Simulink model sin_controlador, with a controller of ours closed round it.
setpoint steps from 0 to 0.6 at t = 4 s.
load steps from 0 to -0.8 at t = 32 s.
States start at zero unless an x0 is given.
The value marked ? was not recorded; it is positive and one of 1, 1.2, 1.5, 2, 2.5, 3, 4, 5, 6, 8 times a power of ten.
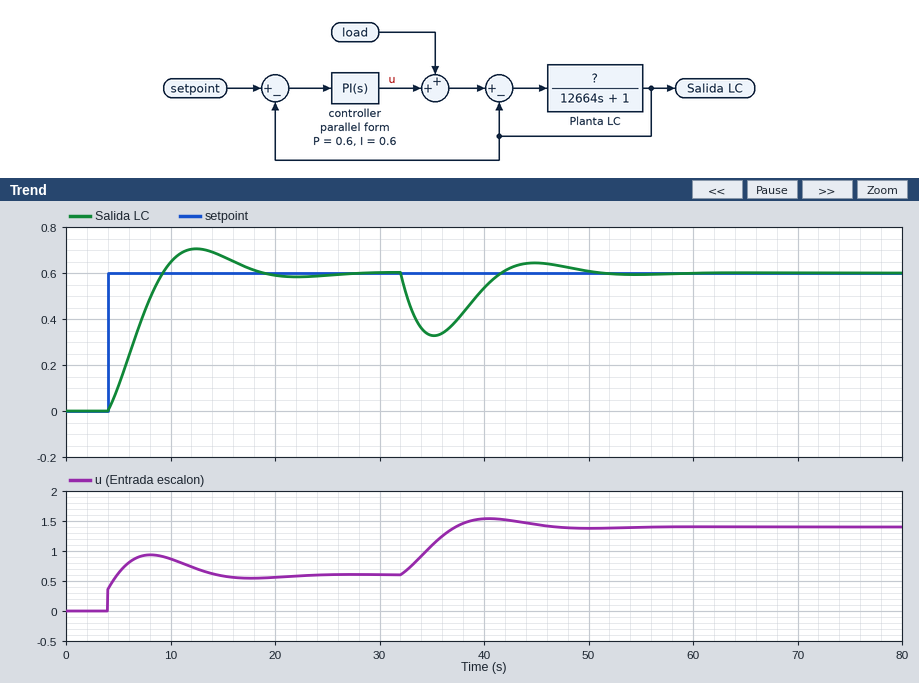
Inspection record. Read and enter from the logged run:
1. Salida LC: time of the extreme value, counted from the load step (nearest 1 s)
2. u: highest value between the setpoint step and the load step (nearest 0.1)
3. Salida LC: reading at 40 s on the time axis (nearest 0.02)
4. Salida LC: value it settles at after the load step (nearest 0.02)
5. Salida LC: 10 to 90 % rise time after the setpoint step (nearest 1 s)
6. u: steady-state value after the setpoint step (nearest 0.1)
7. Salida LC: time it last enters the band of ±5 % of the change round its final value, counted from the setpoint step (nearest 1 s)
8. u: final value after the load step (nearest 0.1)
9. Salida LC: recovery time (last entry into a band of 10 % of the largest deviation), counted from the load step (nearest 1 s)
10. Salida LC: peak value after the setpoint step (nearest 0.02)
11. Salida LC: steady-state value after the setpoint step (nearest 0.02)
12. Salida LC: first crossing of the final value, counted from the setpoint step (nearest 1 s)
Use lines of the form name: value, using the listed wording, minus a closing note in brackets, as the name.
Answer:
Salida LC: time of the extreme value, counted from the load step: 3 s
u: highest value between the setpoint step and the load step: 0.9
Salida LC: reading at 40 s on the time axis: 0.54
Salida LC: value it settles at after the load step: 0.60
Salida LC: 10 to 90 % rise time after the setpoint step: 4 s
u: steady-state value after the setpoint step: 0.6
Salida LC: time it last enters the band of ±5 % of the change round its final value, counted from the setpoint step: 13 s
u: final value after the load step: 1.4
Salida LC: recovery time (last entry into a band of 10 % of the largest deviation), counted from the load step: 16 s
Salida LC: peak value after the setpoint step: 0.70
Salida LC: steady-state value after the setpoint step: 0.60
Salida LC: first crossing of the final value, counted from the setpoint step: 5 s
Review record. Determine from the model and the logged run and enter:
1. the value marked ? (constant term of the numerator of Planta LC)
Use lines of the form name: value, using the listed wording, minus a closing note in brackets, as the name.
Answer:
the value marked ?: 3000
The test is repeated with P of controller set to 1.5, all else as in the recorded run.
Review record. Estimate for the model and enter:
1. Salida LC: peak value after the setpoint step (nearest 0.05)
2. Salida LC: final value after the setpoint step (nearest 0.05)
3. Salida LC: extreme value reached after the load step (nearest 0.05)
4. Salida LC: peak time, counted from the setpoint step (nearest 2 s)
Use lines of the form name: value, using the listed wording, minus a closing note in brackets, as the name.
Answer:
Salida LC: peak value after the setpoint step: 0.65
Salida LC: final value after the setpoint step: 0.60
Salida LC: extreme value reached after the load step: 0.40
Salida LC: peak time, counted from the setpoint step: 8 s
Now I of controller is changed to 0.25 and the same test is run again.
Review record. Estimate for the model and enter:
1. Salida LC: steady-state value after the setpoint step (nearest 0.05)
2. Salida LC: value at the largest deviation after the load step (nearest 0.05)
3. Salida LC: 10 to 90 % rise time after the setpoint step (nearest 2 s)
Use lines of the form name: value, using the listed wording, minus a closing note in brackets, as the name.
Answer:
Salida LC: steady-state value after the setpoint step: 0.60
Salida LC: value at the largest deviation after the load step: 0.25
Salida LC: 10 to 90 % rise time after the setpoint step: 8 s
